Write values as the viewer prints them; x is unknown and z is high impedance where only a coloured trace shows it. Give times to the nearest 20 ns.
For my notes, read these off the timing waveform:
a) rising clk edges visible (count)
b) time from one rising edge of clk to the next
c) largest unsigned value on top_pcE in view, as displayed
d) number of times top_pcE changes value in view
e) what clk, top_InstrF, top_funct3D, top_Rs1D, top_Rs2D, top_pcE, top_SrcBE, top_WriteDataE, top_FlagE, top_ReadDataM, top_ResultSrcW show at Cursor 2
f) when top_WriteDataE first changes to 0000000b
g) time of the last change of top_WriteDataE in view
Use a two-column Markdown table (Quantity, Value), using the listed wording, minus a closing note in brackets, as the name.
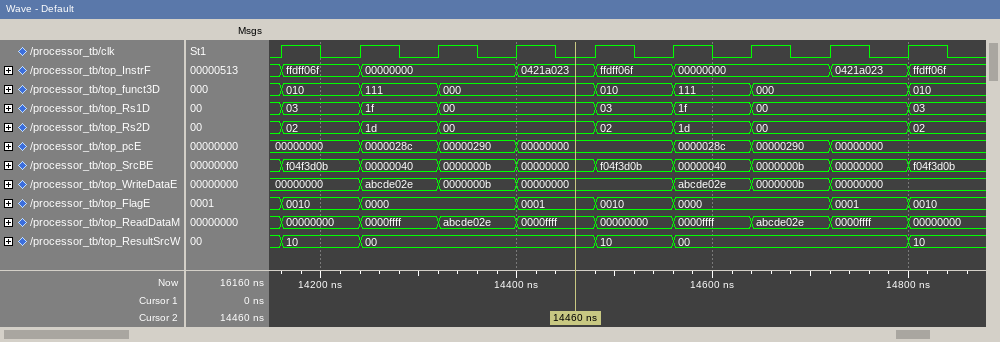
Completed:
| Quantity | Value |
|---|---|
| rising clk edges visible | 9 |
| time from one rising edge of clk to the next | 80 ns |
| largest unsigned value on top_pcE in view, as displayed | 00000290 |
| number of times top_pcE changes value in view | 6 |
| what clk, top_InstrF, top_funct3D, top_Rs1D, top_Rs2D, top_pcE, top_SrcBE, top_WriteDataE, top_FlagE, top_ReadDataM, top_ResultSrcW show at Cursor 2 | clk=0, top_InstrF=0421a023, top_funct3D=000, top_Rs1D=00, top_Rs2D=00, top_pcE=00000000, top_SrcBE=00000000, top_WriteDataE=00000000, top_FlagE=0001, top_ReadDataM=0000ffff, top_ResultSrcW=00 |
| when top_WriteDataE first changes to 0000000b | 14320 ns |
| time of the last change of top_WriteDataE in view | 14720 ns |
